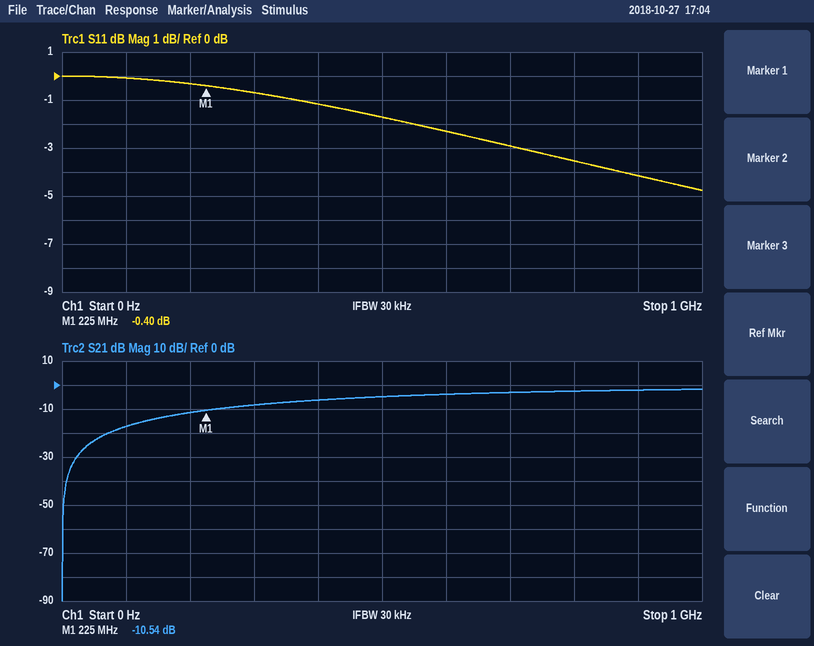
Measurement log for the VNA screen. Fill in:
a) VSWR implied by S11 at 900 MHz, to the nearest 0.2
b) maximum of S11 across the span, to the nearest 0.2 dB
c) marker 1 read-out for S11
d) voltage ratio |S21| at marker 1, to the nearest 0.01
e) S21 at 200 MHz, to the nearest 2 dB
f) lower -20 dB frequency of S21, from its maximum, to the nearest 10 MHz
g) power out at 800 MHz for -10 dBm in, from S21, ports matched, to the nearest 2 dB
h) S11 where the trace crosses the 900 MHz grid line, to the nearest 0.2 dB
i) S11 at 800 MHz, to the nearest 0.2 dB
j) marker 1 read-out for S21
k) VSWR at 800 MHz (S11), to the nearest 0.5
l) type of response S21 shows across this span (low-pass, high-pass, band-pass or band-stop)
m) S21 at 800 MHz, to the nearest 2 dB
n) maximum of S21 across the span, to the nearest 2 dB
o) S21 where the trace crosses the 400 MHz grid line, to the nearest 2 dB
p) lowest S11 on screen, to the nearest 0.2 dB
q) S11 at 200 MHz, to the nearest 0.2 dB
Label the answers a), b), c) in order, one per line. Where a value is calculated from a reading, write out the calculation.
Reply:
a) |Γ| = 10^(-4.2/20) = 0.6166; VSWR = (1 + 0.6166)/(1 − 0.6166) ≈ 4.2
b) 0.0 dB
c) -0.40 dB
d) 10^(-10.54/20) ≈ 0.30
e) -12 dB
f) 60 MHz
g) -10 dBm + (-2 dB) = -12 dBm
h) -4.2 dB
i) -3.6 dB
j) -10.54 dB
k) |Γ| = 10^(-3.6/20) = 0.6607; VSWR = (1 + 0.6607)/(1 − 0.6607) ≈ 4.89, so 5.0 to the nearest 0.5
l) high-pass
m) -2 dB
n) -2 dB
o) -6 dB
p) -4.8 dB
q) -0.4 dB
